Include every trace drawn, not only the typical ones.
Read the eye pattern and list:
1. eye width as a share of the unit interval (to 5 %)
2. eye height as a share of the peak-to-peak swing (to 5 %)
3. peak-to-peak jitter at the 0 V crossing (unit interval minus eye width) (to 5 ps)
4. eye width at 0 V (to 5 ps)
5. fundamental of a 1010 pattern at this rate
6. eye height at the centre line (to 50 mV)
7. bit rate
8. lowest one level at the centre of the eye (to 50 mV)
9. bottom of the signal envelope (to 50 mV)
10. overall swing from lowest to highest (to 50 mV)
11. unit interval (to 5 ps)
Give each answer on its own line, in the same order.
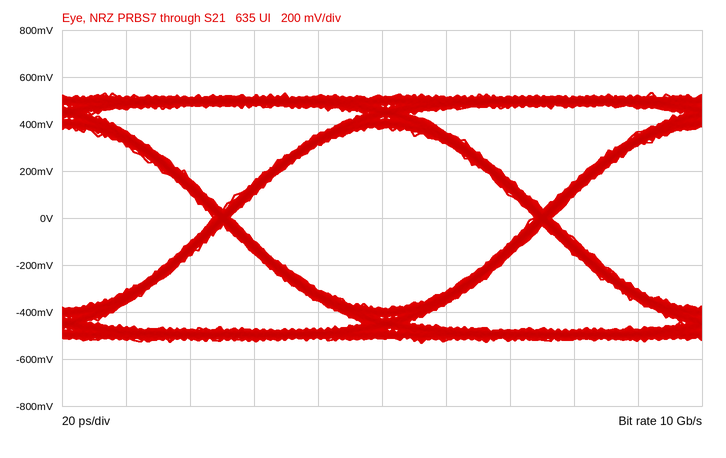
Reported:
95 %
70 %
5 ps
95 ps
5 GHz
750 mV
10 Gb/s
400 mV
-550 mV
1.05 V
100 ps
